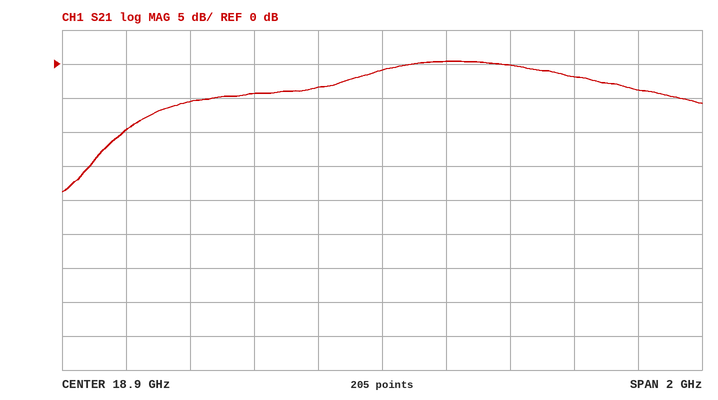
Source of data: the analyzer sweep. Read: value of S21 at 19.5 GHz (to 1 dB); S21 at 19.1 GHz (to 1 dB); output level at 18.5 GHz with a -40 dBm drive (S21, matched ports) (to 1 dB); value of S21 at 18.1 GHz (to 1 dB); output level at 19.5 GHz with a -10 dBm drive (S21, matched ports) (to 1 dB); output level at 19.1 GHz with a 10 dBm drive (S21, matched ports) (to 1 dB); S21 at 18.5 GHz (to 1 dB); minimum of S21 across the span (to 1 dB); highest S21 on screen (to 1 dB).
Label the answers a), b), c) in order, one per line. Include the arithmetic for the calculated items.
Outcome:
a) -2 dB
b) 0 dB
c) -40 dBm + (-4 dB) = -44 dBm
d) -10 dB
e) -10 dBm + (-2 dB) = -12 dBm
f) 10 dBm + (0 dB) = 10 dBm
g) -4 dB
h) -19 dB
i) 0 dB
